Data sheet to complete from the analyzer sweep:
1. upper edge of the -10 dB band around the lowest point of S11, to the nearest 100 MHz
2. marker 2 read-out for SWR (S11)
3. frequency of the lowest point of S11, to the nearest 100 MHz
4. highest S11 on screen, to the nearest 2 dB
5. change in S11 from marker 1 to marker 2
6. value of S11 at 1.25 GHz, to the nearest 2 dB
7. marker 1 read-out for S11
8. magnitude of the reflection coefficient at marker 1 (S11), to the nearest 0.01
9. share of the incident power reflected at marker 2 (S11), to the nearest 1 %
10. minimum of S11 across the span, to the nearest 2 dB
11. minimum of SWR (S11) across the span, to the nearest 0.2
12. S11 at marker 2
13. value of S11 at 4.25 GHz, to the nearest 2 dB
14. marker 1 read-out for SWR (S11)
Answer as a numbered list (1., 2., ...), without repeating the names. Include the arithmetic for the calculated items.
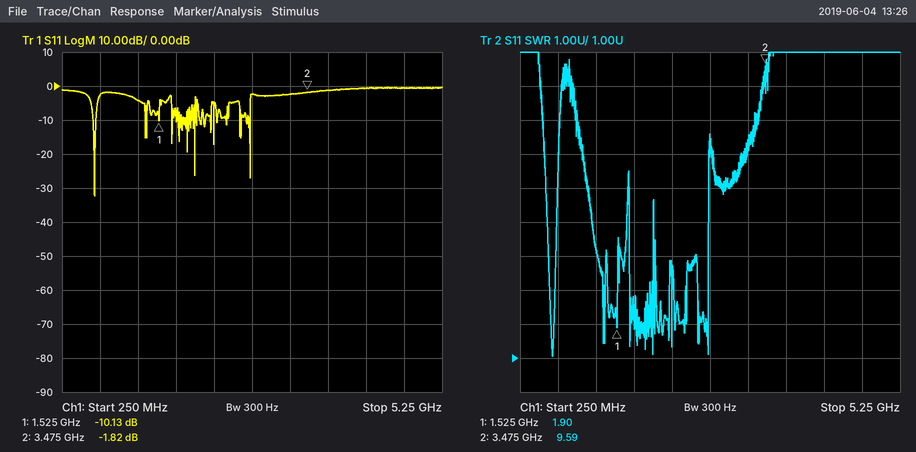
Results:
1. 700 MHz
2. 9.59
3. 700 MHz
4. 0 dB
5. -1.82 − (-10.13) = 8.31 dB
6. -4 dB
7. -10.13 dB
8. 10^(-10.13/20) ≈ 0.31
9. 10^(-1.82/10) ≈ 66 %
10. -32 dB
11. 1.0
12. -1.82 dB
13. 0 dB
14. 1.90
